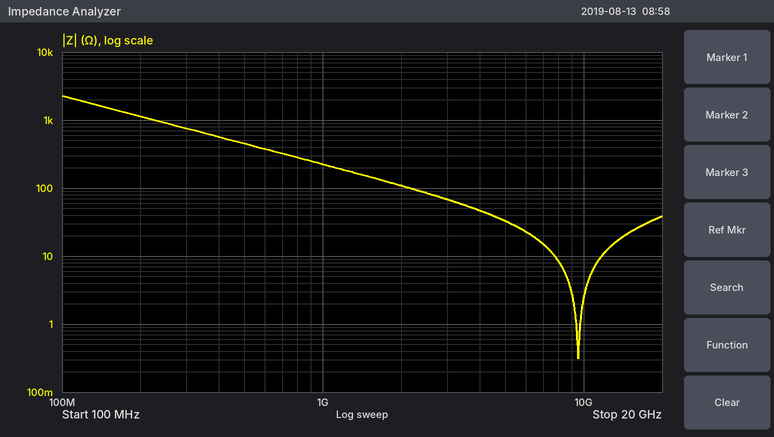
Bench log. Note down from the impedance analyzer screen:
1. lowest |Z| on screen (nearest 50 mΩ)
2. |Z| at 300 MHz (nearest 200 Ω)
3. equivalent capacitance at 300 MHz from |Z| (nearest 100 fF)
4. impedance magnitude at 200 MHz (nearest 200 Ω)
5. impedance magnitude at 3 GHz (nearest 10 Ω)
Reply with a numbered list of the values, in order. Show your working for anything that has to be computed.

1. 300 mΩ
2. 800 Ω
3. C = 1/(2π × 300 MHz × 800 Ω) ≈ 663 fF, so 700 fF to the nearest 100 fF
4. 1.2 kΩ
5. 70 Ω
